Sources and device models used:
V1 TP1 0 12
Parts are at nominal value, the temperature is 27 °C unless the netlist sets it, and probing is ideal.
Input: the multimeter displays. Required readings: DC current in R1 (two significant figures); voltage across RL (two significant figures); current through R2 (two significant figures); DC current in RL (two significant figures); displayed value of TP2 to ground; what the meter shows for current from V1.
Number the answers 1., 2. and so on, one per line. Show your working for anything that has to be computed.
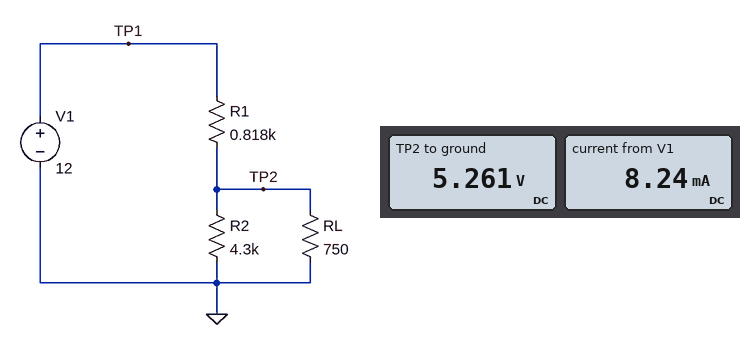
1. (12 V - 5.261 V) / 818 Ω = 8.2 mA
2. 5.261 V = 5.3 V
3. (5.261 V) / 4.3 kΩ = 1.2 mA
4. (5.261 V) / 750 Ω = 7.0 mA
5. 5.261 V
6. 8.24 mA
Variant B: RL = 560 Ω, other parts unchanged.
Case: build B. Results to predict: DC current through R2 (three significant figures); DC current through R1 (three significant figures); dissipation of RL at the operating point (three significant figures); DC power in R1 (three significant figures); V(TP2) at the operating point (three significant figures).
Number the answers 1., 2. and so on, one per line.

1. 1.05 mA
2. 9.14 mA
3. 36.6 mW
4. 68.3 mW
5. 4.53 V
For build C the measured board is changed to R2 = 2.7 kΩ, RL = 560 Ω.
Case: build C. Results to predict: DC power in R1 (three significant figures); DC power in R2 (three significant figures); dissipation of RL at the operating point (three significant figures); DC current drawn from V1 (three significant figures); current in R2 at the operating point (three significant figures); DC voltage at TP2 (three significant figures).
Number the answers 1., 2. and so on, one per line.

1. 71.7 mW
2. 6.98 mW
3. 33.7 mW
4. 9.36 mA
5. 1.61 mA
6. 4.34 V
